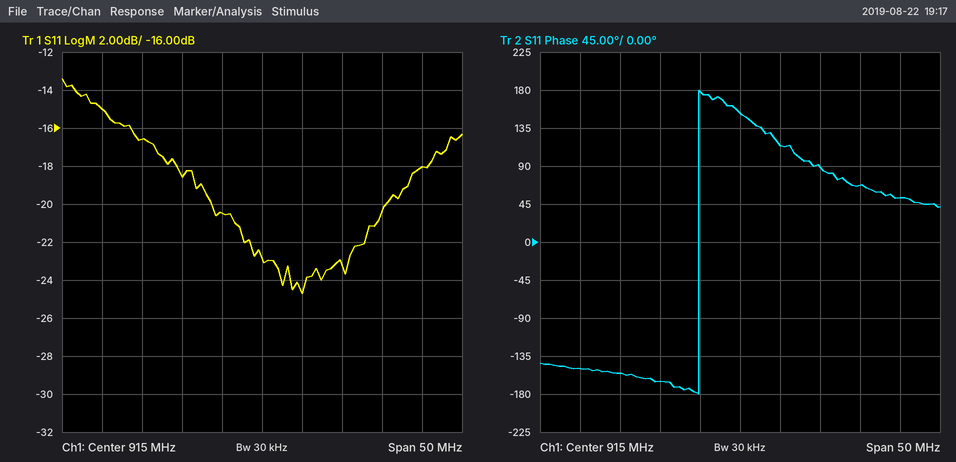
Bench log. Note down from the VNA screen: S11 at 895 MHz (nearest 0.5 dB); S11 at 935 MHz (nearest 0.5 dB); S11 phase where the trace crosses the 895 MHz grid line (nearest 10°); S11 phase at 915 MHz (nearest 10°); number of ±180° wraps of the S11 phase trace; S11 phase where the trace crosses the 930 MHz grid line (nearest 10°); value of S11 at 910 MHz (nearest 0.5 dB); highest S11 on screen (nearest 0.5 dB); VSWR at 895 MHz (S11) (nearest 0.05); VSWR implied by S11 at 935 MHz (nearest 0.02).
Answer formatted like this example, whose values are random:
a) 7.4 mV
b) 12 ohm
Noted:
a) -15.0 dB
b) -18.0 dB
c) -150°
d) 150°
e) 1
f) 70°
g) -20.5 dB
h) -13.5 dB
i) 1.45
j) 1.28
